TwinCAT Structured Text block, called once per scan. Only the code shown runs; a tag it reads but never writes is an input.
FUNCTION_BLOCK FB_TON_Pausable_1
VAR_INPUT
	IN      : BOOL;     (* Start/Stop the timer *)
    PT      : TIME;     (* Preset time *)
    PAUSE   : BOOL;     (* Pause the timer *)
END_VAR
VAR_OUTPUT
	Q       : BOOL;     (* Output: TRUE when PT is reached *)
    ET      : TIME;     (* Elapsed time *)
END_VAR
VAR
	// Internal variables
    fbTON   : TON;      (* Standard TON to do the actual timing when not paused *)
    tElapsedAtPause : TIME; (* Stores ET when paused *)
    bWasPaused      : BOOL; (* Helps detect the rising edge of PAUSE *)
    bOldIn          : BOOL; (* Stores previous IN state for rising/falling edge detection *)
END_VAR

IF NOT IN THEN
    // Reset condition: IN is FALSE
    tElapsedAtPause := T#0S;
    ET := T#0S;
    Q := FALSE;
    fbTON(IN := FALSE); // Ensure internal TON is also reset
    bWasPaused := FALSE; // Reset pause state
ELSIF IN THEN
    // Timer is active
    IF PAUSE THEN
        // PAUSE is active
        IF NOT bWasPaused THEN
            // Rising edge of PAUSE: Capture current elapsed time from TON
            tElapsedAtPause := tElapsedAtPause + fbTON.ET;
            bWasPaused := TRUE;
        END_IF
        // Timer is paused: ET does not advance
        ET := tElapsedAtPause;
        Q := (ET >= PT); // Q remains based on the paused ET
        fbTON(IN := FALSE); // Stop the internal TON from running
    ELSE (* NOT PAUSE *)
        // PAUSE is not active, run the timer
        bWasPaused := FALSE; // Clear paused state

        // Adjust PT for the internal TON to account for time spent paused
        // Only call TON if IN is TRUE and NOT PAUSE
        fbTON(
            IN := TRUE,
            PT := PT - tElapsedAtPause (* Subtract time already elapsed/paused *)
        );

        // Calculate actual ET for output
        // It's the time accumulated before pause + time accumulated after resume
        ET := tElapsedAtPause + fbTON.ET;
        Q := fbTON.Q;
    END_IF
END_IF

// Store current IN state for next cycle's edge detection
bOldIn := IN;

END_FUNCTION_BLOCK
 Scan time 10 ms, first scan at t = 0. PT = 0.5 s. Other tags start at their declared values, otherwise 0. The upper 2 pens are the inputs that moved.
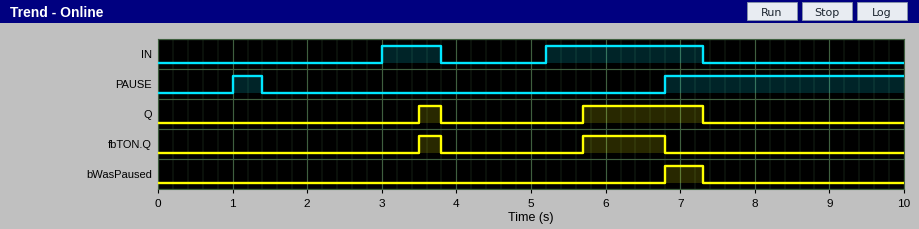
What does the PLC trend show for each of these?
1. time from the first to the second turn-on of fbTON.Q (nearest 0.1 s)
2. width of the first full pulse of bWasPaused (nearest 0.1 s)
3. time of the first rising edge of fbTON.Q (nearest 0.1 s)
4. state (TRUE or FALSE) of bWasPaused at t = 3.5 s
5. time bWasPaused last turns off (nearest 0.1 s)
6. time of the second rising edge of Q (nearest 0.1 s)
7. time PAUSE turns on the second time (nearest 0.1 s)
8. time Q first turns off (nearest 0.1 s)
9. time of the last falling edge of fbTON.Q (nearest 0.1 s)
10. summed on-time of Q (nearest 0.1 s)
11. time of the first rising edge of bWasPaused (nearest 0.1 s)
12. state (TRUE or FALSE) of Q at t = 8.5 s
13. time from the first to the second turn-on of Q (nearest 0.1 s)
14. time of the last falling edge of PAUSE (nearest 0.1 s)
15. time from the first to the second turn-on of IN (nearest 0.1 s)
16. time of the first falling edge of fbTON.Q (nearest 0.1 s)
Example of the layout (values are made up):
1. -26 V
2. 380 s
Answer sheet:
1. 2.2 s
2. 0.5 s
3. 3.5 s
4. FALSE
5. 7.3 s
6. 5.7 s
7. 6.8 s
8. 3.8 s
9. 6.8 s
10. 1.9 s
11. 6.8 s
12. FALSE
13. 2.2 s
14. 1.4 s
15. 2.2 s
16. 3.8 s
